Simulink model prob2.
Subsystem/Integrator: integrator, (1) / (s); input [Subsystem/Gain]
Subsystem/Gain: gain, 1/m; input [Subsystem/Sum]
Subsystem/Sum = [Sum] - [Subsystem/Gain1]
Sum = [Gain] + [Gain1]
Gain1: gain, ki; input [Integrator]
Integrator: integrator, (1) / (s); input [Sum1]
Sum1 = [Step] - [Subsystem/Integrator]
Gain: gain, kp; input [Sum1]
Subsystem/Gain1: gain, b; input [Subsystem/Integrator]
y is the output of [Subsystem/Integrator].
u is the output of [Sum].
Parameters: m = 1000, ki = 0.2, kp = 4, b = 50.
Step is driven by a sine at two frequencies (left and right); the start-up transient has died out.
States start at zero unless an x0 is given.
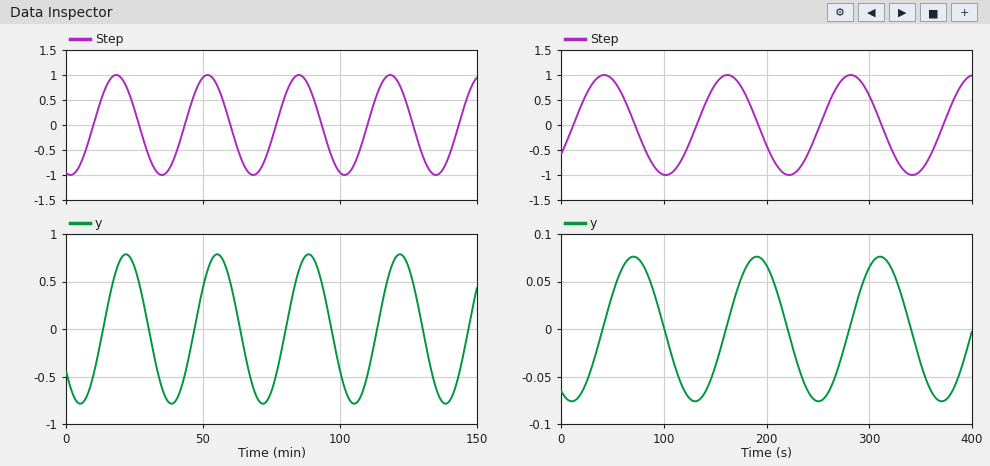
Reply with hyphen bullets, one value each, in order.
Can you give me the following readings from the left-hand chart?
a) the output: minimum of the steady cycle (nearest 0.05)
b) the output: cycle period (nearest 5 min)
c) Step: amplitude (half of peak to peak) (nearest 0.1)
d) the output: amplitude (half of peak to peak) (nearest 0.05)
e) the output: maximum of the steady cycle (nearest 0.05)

- -0.80
- 35 min
- 1.0
- 0.80
- 0.80
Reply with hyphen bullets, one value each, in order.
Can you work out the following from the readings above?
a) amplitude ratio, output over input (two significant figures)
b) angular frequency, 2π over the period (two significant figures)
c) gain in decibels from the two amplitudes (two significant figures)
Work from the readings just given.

- 0.80
- 0.18 rad/min
- -1.9 dB
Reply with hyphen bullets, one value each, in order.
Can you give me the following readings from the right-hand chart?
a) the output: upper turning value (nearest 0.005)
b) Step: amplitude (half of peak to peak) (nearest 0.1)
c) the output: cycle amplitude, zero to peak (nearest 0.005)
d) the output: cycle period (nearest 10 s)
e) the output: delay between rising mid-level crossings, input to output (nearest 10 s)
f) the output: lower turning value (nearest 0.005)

- 0.075
- 1.0
- 0.075
- 120 s
- 30 s
- -0.075
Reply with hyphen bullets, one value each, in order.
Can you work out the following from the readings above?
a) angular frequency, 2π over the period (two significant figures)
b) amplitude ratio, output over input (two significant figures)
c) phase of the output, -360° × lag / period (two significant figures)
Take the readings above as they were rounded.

- 0.052 rad/s
- 0.075
- -90°
